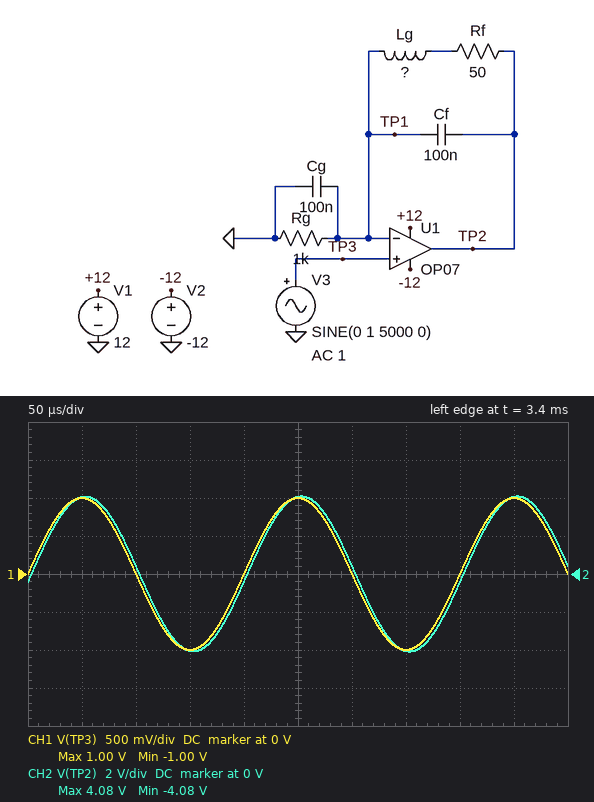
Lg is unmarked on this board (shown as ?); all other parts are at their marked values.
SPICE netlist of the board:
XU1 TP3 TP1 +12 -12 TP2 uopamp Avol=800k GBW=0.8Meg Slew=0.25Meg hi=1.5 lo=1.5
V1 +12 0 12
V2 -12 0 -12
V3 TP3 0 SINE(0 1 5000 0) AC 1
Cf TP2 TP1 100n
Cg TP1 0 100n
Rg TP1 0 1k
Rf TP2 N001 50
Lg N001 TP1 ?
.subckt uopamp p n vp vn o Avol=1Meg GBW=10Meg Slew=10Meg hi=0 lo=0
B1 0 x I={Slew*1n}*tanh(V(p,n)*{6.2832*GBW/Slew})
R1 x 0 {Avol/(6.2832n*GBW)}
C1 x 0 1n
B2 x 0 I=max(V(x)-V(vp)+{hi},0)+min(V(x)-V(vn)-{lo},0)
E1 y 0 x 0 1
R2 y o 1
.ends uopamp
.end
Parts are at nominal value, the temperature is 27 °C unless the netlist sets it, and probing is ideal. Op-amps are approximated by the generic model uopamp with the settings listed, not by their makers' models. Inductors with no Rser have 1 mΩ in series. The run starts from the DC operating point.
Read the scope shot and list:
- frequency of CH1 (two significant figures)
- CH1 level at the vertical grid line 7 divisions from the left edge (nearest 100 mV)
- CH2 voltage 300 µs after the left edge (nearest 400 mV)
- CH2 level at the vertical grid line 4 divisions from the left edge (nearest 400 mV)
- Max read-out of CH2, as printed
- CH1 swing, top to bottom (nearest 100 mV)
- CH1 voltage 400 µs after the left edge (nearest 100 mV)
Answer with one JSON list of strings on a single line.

["5.0 kHz", "-1.0 V", "400 mV", "-400 mV", "4.08 V", "2.0 V", "0 V"]
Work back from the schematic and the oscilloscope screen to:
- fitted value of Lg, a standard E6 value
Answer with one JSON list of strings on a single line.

["15 mH"]
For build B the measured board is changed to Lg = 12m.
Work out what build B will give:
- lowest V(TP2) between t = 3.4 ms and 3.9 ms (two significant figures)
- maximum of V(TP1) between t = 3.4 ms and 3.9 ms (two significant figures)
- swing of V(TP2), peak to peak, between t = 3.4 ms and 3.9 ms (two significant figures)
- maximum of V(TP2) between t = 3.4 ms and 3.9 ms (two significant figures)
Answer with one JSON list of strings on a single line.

["-6.2 V", "1.0 V", "12 V", "6.2 V"]
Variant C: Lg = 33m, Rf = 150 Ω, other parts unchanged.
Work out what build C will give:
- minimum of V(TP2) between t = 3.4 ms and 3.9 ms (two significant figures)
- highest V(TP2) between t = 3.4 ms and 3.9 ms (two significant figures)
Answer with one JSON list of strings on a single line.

["-2.5 V", "2.5 V"]
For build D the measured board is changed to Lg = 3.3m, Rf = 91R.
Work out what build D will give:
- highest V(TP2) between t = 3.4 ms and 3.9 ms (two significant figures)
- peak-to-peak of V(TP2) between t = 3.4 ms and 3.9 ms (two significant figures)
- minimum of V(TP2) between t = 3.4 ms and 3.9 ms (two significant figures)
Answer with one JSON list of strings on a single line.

["1.1 V", "2.2 V", "-1.1 V"]
